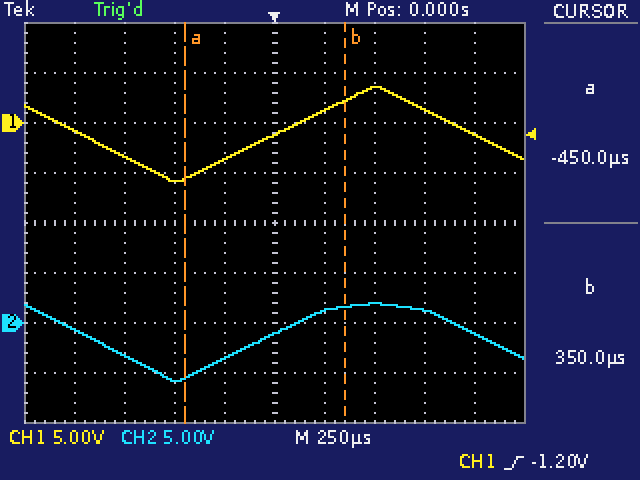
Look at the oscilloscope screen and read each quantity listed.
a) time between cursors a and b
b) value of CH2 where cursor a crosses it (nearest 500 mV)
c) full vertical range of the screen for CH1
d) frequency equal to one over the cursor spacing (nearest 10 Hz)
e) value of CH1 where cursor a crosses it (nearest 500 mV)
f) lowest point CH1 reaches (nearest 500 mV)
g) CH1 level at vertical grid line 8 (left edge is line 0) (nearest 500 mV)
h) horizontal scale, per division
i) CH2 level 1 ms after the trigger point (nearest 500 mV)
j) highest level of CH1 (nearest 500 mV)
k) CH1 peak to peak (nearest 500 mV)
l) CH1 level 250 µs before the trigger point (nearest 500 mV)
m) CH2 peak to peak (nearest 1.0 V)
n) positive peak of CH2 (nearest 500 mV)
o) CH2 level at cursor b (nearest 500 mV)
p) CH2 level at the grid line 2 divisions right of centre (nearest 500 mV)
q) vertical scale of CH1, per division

800 µs
-5.5 V
40 V
1.25 kHz
-5.5 V
-6.0 V
1.5 V
250 µs
-1.0 V
3.5 V
9.5 V
-3.5 V
8.0 V
2.0 V
1.5 V
2.0 V
5 V
